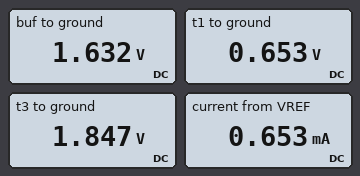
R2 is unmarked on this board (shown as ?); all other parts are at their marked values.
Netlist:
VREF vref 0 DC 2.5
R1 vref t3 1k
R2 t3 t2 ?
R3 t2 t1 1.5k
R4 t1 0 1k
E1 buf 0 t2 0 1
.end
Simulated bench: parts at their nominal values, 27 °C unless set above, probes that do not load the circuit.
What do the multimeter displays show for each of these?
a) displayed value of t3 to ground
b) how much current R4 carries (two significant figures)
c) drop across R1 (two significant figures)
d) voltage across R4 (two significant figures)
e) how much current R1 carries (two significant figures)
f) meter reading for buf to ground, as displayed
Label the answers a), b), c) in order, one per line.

a) 1.847 V
b) 650 µA
c) 650 mV
d) 650 mV
e) 650 µA
f) 1.632 V
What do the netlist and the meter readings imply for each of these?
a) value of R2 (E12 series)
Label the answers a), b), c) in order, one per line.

a) 330 Ω
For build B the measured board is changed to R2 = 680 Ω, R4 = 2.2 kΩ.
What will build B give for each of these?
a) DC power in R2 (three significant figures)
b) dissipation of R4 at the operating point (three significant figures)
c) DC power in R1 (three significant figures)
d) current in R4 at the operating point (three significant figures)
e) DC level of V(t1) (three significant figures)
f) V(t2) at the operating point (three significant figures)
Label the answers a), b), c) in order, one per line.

a) 147 µW
b) 475 µW
c) 216 µW
d) 465 µA
e) 1.02 V
f) 1.72 V
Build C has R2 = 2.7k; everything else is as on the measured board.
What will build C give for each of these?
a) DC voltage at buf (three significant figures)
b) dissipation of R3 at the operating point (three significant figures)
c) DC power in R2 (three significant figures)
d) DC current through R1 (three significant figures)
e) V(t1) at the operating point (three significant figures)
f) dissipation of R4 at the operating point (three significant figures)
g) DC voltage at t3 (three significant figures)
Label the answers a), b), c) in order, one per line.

a) 1.01 V
b) 244 µW
c) 439 µW
d) 403 µA
e) 403 mV
f) 163 µW
g) 2.10 V
